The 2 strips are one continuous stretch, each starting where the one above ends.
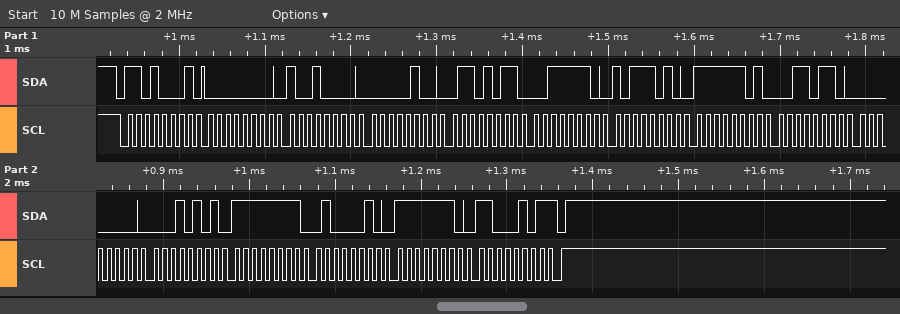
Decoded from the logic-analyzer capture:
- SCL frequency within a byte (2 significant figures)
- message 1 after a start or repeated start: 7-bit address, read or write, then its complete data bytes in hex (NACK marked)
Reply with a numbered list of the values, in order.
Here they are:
1. 100 kHz
2. 0x68 read: 00 90 04 6B 3E BA FD 36 00 15 FF 42 FE C5 NACK
